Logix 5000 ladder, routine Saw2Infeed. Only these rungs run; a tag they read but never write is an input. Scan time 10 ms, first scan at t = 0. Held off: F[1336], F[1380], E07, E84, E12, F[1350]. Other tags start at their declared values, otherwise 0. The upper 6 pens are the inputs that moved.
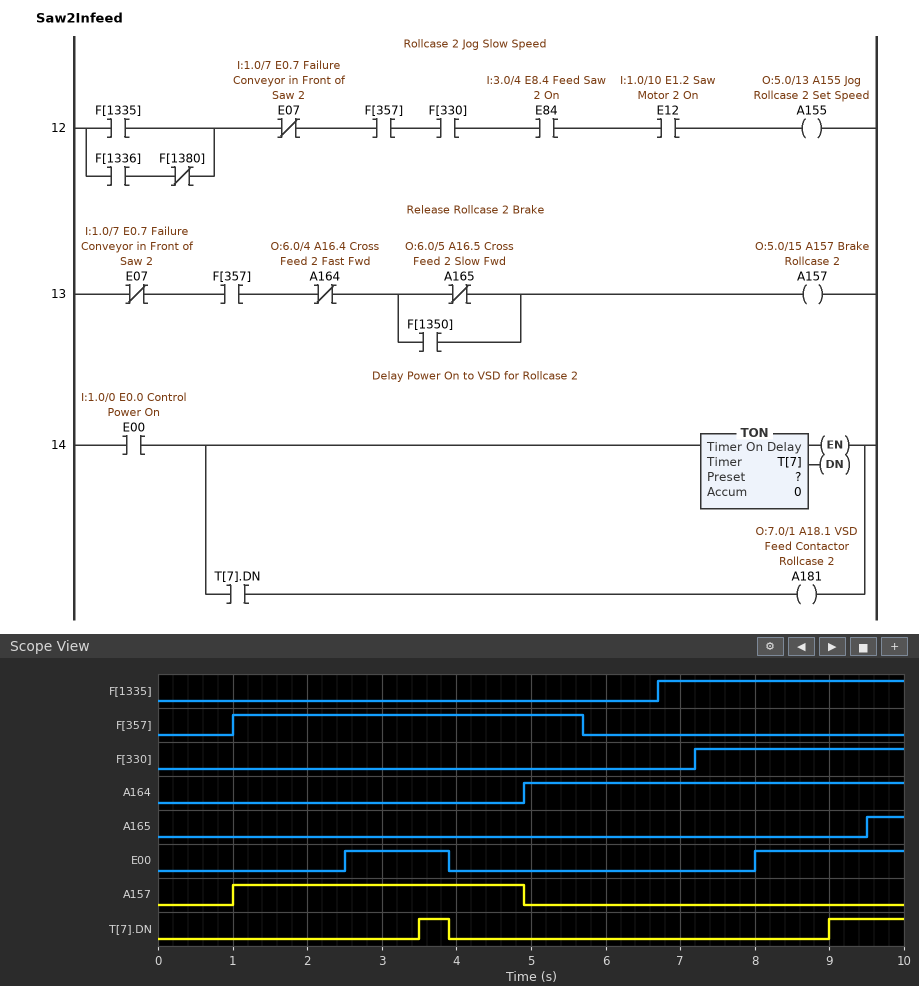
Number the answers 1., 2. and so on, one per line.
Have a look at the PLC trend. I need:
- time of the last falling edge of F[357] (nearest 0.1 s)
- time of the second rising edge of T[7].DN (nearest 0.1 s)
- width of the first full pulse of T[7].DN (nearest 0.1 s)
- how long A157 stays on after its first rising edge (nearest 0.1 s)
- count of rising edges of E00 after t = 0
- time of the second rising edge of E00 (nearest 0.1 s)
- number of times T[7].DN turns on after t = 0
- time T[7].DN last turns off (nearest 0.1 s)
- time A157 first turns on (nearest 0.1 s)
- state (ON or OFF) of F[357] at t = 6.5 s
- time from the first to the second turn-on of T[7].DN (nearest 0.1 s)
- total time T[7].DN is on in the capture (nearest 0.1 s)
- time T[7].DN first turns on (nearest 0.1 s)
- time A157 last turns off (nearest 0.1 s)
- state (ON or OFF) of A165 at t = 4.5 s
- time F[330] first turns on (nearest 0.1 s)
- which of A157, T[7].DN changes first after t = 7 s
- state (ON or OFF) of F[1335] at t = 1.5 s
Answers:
1. 5.7 s
2. 9.0 s
3. 0.4 s
4. 3.9 s
5. 2
6. 8.0 s
7. 2
8. 3.9 s
9. 1.0 s
10. OFF
11. 5.5 s
12. 1.4 s
13. 3.5 s
14. 4.9 s
15. OFF
16. 7.2 s
17. T[7].DN
18. OFF
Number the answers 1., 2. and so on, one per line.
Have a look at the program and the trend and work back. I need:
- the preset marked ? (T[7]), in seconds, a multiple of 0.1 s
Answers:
1. 1.0 s
